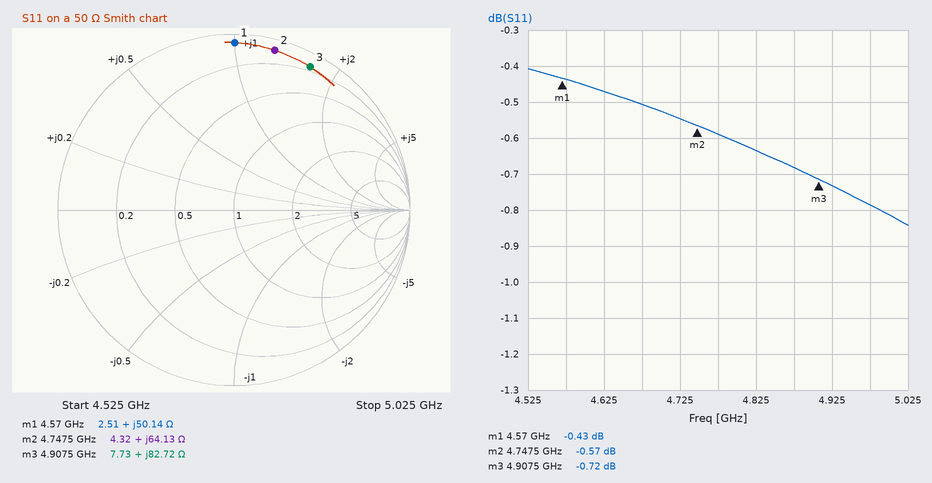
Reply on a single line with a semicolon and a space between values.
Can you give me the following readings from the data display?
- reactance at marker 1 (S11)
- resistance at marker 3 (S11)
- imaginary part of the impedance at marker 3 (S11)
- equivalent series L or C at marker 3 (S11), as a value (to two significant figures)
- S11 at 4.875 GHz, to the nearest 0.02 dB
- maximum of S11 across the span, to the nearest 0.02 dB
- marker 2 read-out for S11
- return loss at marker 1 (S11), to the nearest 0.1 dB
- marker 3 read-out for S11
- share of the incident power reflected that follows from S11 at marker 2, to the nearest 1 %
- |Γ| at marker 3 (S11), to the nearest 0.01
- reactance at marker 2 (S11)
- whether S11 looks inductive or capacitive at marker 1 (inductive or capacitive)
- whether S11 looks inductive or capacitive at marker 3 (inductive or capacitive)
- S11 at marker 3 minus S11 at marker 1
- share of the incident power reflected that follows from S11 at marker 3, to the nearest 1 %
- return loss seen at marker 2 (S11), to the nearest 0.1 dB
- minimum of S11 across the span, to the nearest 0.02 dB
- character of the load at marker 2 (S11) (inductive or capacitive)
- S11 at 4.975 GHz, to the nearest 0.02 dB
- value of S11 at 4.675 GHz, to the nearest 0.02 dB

+50.14 Ω; 7.73 Ω; +82.72 Ω; 2.7 nH; -0.68 dB; -0.40 dB; -0.57 dB; 0.4 dB; -0.72 dB; 88 %; 0.92; +64.13 Ω; inductive; inductive; -0.29 dB; 85 %; 0.6 dB; -0.84 dB; inductive; -0.78 dB; -0.50 dB
